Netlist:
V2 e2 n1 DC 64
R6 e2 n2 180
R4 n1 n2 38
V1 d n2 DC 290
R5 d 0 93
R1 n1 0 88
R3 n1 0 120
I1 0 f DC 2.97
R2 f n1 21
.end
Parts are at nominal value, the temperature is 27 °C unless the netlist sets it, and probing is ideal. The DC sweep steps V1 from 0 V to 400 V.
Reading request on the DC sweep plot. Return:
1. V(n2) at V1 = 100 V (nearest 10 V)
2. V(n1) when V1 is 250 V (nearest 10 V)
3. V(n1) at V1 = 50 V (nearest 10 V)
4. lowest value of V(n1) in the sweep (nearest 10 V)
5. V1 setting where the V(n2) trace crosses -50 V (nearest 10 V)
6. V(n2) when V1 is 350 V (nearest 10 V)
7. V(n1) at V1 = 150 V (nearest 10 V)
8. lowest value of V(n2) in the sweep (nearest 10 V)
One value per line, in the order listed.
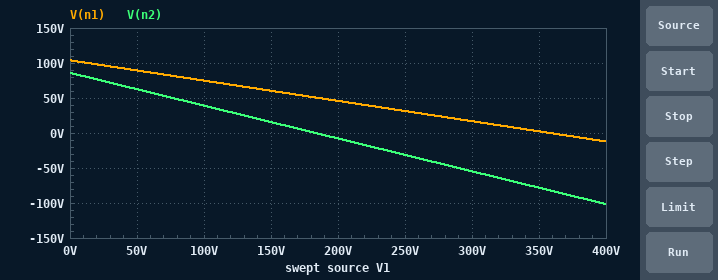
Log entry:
40 V
30 V
90 V
-10 V
290 V
-80 V
60 V
-100 V
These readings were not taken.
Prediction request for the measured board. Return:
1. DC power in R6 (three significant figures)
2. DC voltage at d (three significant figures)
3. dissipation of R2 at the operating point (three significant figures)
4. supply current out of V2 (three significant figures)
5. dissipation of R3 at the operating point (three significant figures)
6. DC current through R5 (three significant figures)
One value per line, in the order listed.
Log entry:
99.5 W
240 V
185 W
743 mA
3.26 W
2.58 A
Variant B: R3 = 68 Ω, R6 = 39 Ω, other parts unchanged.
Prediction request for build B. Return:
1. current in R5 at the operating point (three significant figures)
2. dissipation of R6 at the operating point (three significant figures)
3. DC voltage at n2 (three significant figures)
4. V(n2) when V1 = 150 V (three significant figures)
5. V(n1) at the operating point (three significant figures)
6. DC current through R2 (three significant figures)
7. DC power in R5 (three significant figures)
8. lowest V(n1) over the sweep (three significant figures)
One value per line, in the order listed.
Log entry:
2.89 A
199 W
-21.1 V
32.5 V
3.00 V
2.97 A
778 W
-25.0 V
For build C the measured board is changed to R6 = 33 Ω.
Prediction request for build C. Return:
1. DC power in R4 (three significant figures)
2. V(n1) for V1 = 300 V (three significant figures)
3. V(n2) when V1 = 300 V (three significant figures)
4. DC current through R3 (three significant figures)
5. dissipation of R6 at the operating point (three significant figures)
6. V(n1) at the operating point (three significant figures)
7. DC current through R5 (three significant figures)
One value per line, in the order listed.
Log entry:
8.26 W
-1.76 V
-20.6 V
11.6 mA
202 W
1.39 V
2.94 A
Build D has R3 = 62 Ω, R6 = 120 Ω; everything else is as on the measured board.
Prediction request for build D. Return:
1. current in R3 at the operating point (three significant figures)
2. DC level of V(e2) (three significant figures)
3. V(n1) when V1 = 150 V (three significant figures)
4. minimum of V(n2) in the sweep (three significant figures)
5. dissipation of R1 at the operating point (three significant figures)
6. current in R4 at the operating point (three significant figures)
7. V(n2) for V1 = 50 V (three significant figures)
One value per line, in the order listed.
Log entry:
210 mA
77.0 V
45.2 V
-92.4 V
1.92 W
1.58 A
51.9 V
